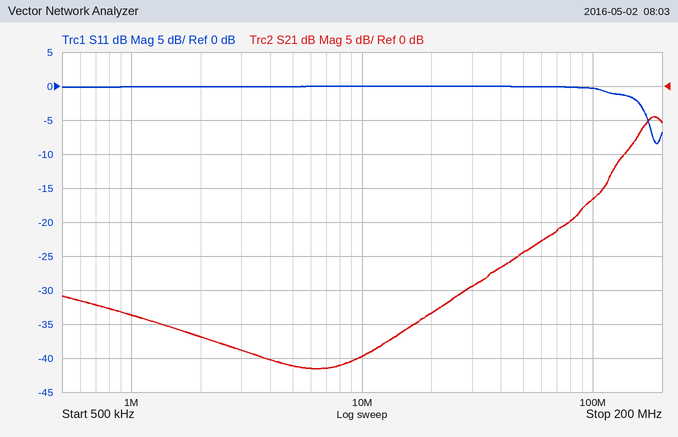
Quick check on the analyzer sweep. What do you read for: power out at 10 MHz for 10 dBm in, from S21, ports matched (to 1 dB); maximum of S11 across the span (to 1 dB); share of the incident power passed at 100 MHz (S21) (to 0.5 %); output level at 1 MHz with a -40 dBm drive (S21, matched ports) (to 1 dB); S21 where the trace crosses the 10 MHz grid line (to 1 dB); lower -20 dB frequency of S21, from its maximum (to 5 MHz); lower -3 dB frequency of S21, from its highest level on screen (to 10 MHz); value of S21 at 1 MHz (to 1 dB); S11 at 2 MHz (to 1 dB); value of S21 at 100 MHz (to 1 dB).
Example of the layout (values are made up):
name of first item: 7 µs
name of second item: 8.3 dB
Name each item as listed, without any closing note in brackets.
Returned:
power out at 10 MHz for 10 dBm in, from S21, ports matched: -30 dBm
maximum of S11 across the span: 0 dB
share of the incident power passed at 100 MHz (S21): 2.0 %
output level at 1 MHz with a -40 dBm drive (S21, matched ports): -74 dBm
S21 where the trace crosses the 10 MHz grid line: -40 dB
lower -20 dB frequency of S21, from its maximum: 50 MHz
lower -3 dB frequency of S21, from its highest level on screen: 160 MHz
value of S21 at 1 MHz: -34 dB
S11 at 2 MHz: 0 dB
value of S21 at 100 MHz: -17 dB
